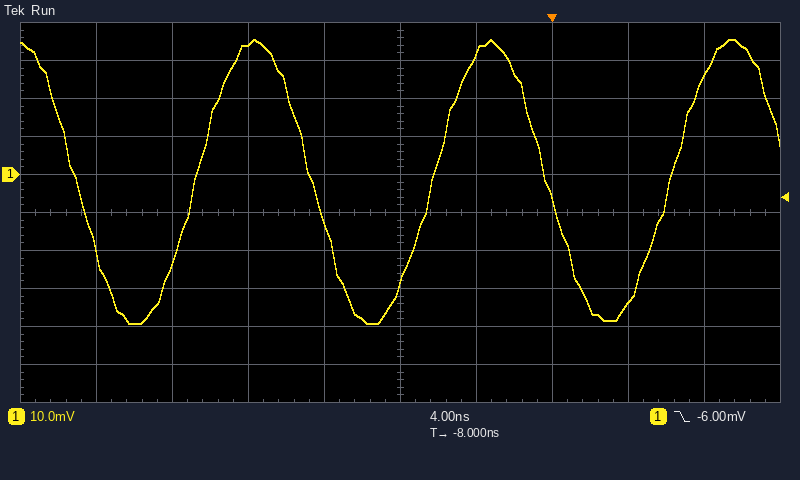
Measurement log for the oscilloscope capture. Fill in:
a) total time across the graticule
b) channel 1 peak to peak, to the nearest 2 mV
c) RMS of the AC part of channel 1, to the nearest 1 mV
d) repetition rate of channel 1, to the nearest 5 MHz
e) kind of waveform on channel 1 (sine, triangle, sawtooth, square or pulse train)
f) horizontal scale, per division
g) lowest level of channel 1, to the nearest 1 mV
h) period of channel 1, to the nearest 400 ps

40 ns
74 mV
26 mV
80 MHz
sine
4 ns
-39 mV
12.4 ns
